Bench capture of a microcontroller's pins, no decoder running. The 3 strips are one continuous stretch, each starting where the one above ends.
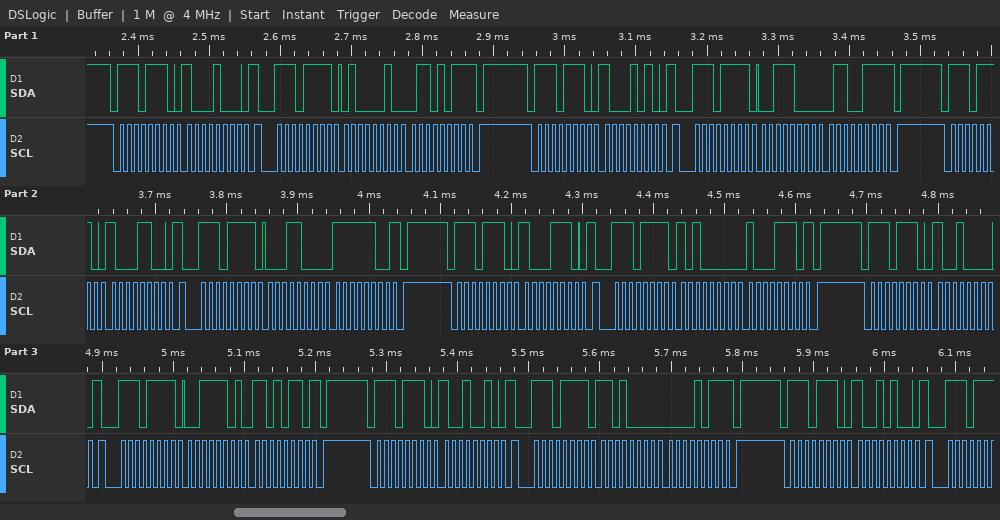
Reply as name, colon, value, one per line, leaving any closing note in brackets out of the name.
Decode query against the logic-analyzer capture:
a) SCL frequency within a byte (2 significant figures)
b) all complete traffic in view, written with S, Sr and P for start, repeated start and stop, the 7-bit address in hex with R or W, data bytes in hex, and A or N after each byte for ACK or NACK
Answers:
SCL frequency within a byte: 100 kHz
all complete traffic in view, written with S, Sr and P for start, repeated start and stop, the 7-bit address in hex with R or W, data bytes in hex, and A or N after each byte for ACK or NACK: S 77W A 88 A Sr 77R A 42 A 6B N P S 77W A 8A A Sr 77R A 38 A 67 N P S 77W A 8C A Sr 77R A 18 A FC N P S 77W A 8E A Sr 77R A A0 A 8E N P S 77W A 90 A Sr 77R A 3D A D6 N P S 77W A 92 A Sr 77R A D0 A 0B N P S 77W A 94 A
